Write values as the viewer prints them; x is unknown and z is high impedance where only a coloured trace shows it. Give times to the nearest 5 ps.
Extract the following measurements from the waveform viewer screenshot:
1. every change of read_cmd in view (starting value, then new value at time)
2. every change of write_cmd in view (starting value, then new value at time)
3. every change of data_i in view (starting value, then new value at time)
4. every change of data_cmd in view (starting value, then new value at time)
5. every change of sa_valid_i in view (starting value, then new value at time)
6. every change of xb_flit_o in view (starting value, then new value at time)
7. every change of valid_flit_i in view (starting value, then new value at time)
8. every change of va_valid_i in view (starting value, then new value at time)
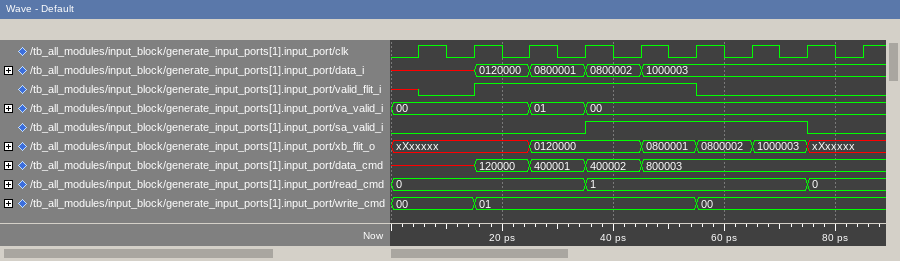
0, 1 at 35 ps, 0 at 75 ps
00, 01 at 15 ps, 00 at 55 ps
x, 0120000 at 15 ps, 0800001 at 25 ps, 0800002 at 35 ps, 1000003 at 45 ps
x, 120000 at 15 ps, 400001 at 25 ps, 400002 at 35 ps, 800003 at 45 ps
0, 1 at 35 ps, 0 at 75 ps
xXxxxxx, 0120000 at 25 ps, 0800001 at 45 ps, 0800002 at 55 ps, 1000003 at 65 ps, xXxxxxx at 75 ps
x, 0 at 5 ps, 1 at 15 ps, 0 at 55 ps
00, 01 at 25 ps, 00 at 35 ps
